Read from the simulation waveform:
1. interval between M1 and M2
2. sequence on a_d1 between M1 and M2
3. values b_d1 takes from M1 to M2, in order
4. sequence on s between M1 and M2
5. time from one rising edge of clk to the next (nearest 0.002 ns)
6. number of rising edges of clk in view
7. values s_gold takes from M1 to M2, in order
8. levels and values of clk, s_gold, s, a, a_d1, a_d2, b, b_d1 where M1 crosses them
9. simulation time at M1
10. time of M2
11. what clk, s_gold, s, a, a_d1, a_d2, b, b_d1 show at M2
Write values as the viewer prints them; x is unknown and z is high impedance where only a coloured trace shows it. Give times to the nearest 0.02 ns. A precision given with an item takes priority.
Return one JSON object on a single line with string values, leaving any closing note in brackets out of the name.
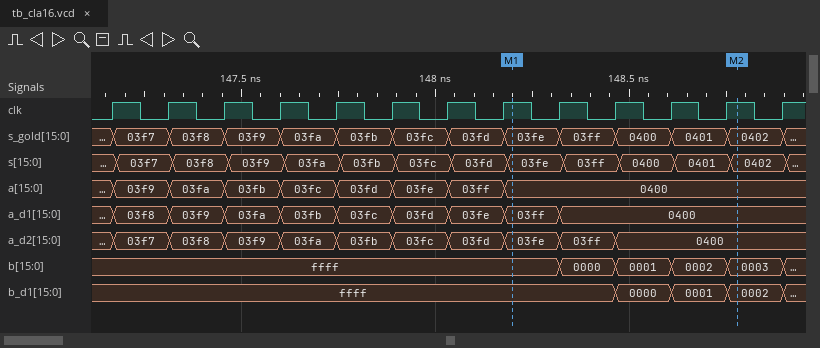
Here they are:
{"interval between M1 and M2": "0.58 ns", "sequence on a_d1 between M1 and M2": "03ff, 0400", "values b_d1 takes from M1 to M2, in order": "ffff, 0000, 0001, 0002", "sequence on s between M1 and M2": "03fe, 03ff, 0400, 0401, 0402", "time from one rising edge of clk to the next": "0.144 ns", "number of rising edges of clk in view": "13", "values s_gold takes from M1 to M2, in order": "03fe, 03ff, 0400, 0401, 0402", "levels and values of clk, s_gold, s, a, a_d1, a_d2, b, b_d1 where M1 crosses them": "clk=1, s_gold=03fe, s=03fe, a=0400, a_d1=03ff, a_d2=03fe, b=ffff, b_d1=ffff", "simulation time at M1": "148.2 ns", "time of M2": "148.78 ns", "what clk, s_gold, s, a, a_d1, a_d2, b, b_d1 show at M2": "clk=1, s_gold=0402, s=0402, a=0400, a_d1=0400, a_d2=0400, b=0003, b_d1=0002"}
